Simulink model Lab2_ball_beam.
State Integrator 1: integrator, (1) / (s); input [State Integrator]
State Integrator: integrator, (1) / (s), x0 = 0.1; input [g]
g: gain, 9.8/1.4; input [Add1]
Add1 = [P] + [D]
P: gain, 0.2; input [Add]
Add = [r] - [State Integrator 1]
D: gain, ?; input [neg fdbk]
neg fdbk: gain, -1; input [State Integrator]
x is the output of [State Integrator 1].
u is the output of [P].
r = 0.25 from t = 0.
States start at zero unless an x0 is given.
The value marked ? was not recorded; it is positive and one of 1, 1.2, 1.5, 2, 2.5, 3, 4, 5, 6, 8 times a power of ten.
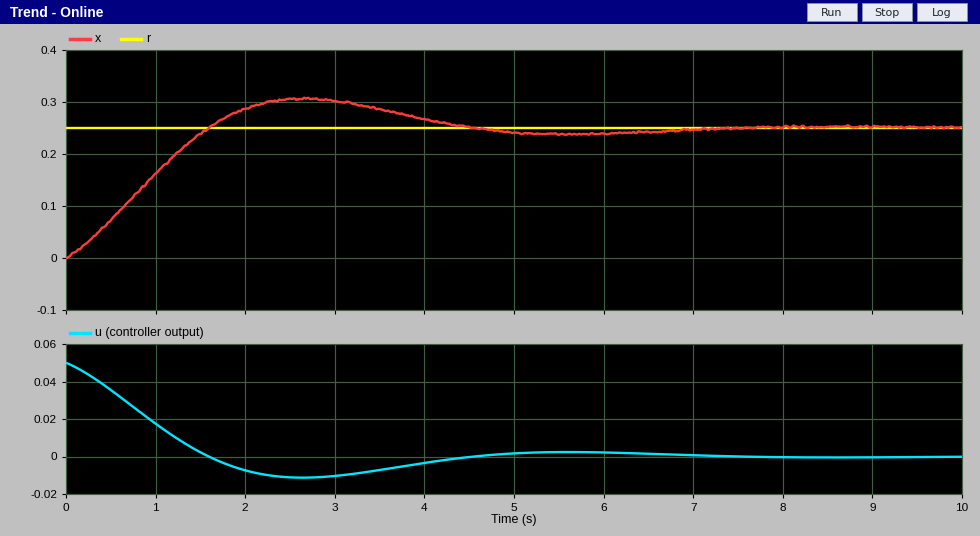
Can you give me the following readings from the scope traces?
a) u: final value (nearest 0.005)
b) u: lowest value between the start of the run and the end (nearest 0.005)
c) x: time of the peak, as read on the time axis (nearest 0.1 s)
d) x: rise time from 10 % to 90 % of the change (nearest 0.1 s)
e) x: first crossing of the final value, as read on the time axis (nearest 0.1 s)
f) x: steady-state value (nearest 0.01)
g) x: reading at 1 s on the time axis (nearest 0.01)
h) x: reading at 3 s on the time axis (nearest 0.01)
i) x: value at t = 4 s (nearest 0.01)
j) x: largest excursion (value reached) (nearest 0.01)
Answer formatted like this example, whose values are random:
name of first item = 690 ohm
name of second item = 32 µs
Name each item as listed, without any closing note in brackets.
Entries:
u: final value = 0.000
u: lowest value between the start of the run and the end = -0.010
x: time of the peak, as read on the time axis = 2.6 s
x: rise time from 10 % to 90 % of the change = 1.2 s
x: first crossing of the final value, as read on the time axis = 1.6 s
x: steady-state value = 0.25
x: reading at 1 s on the time axis = 0.16
x: reading at 3 s on the time axis = 0.30
x: value at t = 4 s = 0.27
x: largest excursion (value reached) = 0.31
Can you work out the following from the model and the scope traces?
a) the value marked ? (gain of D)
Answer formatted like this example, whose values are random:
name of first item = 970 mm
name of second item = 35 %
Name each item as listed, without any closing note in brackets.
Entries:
the value marked ? = 0.15
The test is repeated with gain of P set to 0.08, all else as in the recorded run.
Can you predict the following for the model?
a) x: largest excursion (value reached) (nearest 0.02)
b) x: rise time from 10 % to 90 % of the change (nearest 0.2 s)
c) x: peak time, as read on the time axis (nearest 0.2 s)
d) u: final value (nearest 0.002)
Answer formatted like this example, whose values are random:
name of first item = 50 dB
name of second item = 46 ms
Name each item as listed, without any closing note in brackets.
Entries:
x: largest excursion (value reached) = 0.26
x: rise time from 10 % to 90 % of the change = 2.4 s
x: peak time, as read on the time axis = 4.8 s
u: final value = 0.000
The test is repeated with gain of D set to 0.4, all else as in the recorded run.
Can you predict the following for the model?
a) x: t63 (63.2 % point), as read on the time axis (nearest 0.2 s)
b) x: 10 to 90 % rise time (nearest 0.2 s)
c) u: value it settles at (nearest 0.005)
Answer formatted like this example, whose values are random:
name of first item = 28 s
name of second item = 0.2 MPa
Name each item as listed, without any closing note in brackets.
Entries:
x: t63 (63.2 % point), as read on the time axis = 1.8 s
x: 10 to 90 % rise time = 3.6 s
u: value it settles at = 0.000
